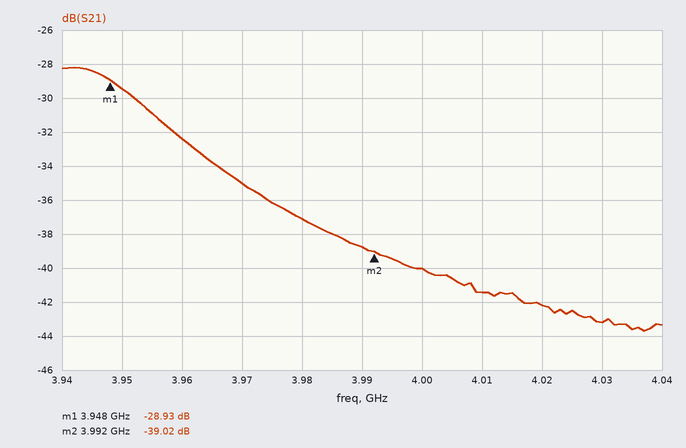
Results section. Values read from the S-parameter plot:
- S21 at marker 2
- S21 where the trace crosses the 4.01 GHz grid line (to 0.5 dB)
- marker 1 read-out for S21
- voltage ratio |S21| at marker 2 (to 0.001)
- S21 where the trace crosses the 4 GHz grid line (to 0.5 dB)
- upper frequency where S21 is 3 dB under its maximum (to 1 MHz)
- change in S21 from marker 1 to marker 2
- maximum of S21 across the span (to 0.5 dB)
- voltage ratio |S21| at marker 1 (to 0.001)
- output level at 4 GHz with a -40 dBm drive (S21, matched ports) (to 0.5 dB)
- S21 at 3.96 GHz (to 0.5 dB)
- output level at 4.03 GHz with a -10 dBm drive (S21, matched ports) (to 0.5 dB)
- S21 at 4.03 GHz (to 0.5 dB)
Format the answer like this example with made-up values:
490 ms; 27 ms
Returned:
-39.02 dB; -41.5 dB; -28.93 dB; 0.011; -40.0 dB; 3.956 GHz; -10.09 dB; -28.0 dB; 0.036; -80.0 dBm; -32.5 dB; -53.0 dBm; -43.0 dB
